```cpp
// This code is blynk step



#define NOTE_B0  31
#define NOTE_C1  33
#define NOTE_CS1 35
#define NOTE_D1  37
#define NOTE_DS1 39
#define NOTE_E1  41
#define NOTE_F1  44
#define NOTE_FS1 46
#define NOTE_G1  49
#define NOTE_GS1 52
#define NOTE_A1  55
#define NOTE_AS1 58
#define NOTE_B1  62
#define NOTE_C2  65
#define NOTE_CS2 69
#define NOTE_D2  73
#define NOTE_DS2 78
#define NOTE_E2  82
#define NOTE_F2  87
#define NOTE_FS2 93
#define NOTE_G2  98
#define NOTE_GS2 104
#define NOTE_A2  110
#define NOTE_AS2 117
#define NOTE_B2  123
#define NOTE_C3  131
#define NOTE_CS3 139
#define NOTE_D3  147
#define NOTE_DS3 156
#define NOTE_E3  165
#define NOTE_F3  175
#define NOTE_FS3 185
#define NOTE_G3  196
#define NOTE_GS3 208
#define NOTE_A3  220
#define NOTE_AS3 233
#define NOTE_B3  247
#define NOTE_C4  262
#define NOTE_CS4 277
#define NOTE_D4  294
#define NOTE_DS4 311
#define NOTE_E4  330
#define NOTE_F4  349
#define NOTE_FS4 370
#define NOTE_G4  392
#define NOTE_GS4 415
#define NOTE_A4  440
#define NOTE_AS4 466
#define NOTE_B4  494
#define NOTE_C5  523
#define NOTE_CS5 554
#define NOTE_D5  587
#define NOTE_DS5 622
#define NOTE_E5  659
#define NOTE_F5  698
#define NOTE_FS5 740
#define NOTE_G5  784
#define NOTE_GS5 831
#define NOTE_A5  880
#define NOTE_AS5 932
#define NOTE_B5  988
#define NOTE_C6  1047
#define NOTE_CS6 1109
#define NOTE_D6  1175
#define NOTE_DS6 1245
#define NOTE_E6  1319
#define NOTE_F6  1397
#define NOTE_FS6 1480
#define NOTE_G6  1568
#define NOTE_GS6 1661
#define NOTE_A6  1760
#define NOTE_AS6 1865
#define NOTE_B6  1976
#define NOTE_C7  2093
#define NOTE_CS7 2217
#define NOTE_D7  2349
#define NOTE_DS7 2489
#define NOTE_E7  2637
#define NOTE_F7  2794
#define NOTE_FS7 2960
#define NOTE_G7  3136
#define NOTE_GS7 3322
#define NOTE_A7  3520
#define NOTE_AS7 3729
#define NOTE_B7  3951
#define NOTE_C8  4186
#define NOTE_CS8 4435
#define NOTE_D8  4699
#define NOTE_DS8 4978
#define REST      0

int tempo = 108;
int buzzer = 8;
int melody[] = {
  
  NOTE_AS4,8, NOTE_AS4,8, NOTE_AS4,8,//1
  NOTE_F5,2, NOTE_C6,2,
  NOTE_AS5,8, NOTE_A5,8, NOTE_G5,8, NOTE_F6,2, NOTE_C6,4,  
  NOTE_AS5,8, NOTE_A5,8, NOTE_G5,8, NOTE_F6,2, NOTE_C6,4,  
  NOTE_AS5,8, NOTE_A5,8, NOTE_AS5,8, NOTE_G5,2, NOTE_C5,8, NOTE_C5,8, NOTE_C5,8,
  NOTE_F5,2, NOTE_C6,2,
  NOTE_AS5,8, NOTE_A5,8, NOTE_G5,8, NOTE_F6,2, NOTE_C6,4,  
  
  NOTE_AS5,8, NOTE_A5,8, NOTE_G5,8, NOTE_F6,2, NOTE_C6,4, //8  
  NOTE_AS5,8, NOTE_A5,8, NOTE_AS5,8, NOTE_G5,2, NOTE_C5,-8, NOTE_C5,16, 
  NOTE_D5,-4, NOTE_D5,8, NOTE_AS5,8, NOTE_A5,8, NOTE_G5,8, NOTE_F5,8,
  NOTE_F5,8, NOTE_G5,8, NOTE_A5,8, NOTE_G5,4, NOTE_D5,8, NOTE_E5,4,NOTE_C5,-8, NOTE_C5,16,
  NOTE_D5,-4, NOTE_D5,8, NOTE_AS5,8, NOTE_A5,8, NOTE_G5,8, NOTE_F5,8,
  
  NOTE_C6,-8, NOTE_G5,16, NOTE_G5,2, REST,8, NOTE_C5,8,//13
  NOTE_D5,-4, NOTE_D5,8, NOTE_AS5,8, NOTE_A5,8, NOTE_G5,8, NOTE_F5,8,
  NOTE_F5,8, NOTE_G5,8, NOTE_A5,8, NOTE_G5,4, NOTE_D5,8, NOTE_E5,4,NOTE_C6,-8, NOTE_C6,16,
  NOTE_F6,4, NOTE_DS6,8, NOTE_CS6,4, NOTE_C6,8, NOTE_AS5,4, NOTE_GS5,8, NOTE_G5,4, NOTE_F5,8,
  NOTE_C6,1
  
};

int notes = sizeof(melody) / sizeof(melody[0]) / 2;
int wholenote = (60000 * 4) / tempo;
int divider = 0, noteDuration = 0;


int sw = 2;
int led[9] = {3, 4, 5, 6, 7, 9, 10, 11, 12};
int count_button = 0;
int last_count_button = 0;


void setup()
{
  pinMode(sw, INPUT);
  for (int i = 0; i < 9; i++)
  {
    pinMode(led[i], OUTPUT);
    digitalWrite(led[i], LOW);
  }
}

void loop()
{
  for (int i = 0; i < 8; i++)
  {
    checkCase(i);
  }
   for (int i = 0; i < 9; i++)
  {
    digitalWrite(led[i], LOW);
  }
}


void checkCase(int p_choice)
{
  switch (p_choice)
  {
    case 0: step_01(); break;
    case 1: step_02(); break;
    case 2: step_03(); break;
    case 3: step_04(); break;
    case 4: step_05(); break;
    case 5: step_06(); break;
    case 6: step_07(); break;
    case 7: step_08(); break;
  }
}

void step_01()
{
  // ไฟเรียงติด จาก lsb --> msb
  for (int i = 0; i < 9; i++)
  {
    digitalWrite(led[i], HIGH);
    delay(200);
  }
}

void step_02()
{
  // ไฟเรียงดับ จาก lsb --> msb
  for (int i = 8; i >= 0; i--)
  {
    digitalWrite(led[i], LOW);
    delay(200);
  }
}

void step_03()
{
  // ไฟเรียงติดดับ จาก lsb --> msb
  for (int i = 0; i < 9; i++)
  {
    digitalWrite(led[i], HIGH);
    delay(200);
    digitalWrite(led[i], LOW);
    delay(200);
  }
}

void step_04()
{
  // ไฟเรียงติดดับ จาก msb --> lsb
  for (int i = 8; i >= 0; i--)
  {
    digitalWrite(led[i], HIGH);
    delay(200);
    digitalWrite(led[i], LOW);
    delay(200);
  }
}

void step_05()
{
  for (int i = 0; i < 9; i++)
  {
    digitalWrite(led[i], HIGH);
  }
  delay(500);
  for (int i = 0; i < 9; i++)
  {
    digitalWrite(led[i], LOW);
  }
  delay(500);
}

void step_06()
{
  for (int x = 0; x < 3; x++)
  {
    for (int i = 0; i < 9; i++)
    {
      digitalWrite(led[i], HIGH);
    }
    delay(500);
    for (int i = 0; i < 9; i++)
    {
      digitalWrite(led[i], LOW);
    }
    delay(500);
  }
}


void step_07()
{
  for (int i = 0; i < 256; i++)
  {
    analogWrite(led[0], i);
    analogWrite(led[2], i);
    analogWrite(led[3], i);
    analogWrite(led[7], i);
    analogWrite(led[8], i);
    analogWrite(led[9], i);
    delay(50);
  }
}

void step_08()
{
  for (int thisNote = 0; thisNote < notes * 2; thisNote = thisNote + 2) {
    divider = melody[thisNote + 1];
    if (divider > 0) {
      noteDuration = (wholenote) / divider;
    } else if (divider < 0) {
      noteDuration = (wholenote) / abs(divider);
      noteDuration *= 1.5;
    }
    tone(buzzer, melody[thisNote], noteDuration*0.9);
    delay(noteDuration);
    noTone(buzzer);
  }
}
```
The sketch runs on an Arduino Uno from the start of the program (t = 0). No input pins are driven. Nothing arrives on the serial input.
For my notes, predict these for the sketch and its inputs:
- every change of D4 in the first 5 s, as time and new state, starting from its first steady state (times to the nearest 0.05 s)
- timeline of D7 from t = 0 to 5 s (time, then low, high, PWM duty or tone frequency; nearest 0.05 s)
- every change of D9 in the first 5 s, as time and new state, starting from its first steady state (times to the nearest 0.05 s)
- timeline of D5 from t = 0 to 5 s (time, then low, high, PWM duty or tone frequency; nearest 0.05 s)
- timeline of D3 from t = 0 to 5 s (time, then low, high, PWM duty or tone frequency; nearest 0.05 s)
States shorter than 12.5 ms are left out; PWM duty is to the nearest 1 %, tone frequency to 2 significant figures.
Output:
0 s low; 0.2 s high; 3.2 s low; 4 s high; 4.2 s low
0 s low; 0.8 s high; 2.6 s low
0 s low; 1 s high; 2.4 s low
0 s low; 0.4 s high; 3 s low; 4.4 s high; 4.6 s low
0 s high; 3.4 s low; 3.6 s high; 3.8 s low
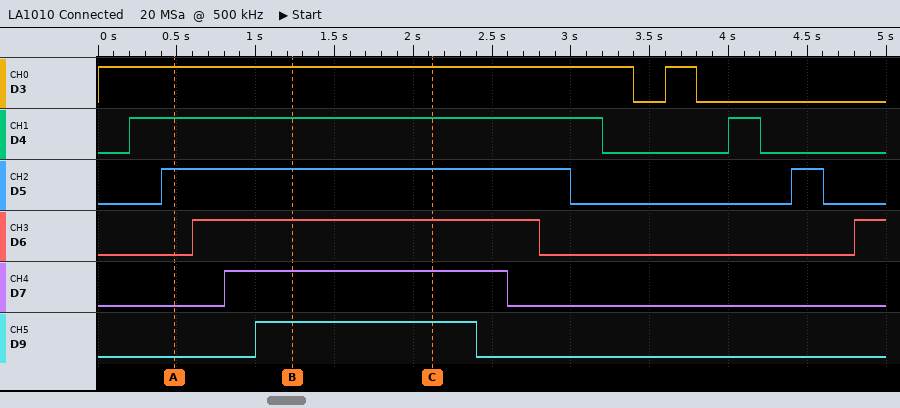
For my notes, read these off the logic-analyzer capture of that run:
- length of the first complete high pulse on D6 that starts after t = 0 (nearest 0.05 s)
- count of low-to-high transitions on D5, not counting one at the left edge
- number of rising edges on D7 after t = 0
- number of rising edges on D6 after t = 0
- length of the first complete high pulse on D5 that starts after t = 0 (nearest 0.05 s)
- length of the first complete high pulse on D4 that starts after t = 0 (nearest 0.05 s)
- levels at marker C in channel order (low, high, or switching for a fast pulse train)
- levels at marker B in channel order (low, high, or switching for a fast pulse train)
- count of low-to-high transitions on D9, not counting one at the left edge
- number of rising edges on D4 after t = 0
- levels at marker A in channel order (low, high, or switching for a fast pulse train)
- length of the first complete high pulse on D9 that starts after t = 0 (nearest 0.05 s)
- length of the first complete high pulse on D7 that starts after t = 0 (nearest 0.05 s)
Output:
2.20 s
2
1
2
2.60 s
3.00 s
D3 high, D4 high, D5 high, D6 high, D7 high, D9 high
D3 high, D4 high, D5 high, D6 high, D7 high, D9 high
1
2
D3 high, D4 high, D5 high, D6 low, D7 low, D9 low
1.40 s
1.80 s
